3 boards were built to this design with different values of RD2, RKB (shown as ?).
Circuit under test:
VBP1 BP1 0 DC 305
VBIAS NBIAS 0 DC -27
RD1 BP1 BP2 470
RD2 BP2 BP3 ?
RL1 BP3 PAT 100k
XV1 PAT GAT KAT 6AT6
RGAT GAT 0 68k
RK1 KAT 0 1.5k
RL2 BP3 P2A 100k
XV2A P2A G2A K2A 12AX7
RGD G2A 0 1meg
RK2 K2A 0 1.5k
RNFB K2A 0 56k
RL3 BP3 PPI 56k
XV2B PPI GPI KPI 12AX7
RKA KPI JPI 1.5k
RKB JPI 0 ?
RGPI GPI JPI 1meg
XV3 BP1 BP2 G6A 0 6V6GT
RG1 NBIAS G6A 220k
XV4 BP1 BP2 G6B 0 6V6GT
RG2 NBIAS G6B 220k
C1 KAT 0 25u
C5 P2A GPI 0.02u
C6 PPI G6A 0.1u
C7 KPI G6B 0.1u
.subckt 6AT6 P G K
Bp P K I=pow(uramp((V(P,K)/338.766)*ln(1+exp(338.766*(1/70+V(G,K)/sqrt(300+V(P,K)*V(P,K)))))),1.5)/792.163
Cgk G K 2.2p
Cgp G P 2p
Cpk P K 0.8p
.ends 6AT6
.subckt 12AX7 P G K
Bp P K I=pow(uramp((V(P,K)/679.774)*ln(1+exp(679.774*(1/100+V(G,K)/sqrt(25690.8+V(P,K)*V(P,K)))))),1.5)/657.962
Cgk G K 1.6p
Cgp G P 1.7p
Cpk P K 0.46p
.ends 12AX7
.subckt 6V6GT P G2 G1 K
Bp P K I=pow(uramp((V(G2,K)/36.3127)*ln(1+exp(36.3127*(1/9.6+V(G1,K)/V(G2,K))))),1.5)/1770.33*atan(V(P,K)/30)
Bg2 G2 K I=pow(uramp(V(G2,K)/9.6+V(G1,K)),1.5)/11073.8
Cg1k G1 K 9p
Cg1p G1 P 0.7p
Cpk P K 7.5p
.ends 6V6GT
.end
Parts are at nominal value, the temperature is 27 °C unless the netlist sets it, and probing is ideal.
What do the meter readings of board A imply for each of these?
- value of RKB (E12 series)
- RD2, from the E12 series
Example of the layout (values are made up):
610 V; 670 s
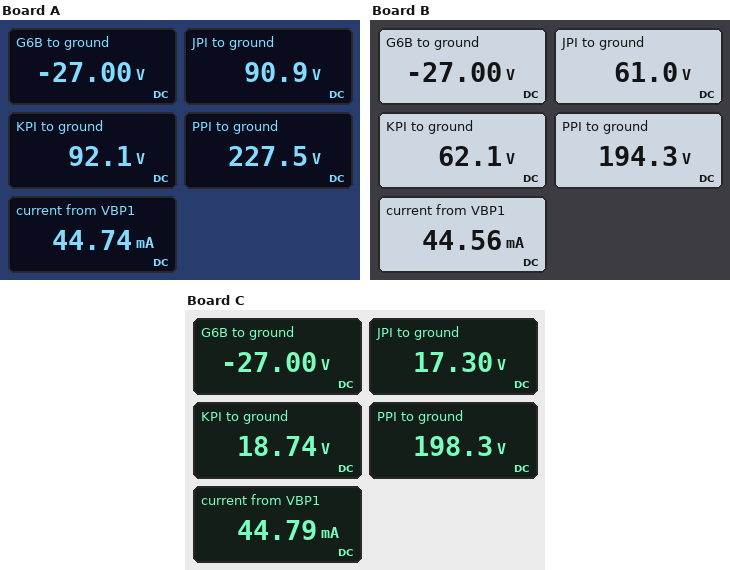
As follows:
120 kΩ; 12 kΩ
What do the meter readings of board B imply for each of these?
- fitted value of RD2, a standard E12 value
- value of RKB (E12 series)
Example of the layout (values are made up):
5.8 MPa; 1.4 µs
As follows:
27 kΩ; 82 kΩ
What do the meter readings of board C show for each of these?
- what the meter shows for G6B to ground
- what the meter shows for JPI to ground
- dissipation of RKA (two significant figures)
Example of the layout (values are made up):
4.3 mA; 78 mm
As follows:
-27.00 V; 17.30 V; 1.4 mW
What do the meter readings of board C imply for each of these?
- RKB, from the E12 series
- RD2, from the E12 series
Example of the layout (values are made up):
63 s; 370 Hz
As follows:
18 kΩ; 18 kΩ
